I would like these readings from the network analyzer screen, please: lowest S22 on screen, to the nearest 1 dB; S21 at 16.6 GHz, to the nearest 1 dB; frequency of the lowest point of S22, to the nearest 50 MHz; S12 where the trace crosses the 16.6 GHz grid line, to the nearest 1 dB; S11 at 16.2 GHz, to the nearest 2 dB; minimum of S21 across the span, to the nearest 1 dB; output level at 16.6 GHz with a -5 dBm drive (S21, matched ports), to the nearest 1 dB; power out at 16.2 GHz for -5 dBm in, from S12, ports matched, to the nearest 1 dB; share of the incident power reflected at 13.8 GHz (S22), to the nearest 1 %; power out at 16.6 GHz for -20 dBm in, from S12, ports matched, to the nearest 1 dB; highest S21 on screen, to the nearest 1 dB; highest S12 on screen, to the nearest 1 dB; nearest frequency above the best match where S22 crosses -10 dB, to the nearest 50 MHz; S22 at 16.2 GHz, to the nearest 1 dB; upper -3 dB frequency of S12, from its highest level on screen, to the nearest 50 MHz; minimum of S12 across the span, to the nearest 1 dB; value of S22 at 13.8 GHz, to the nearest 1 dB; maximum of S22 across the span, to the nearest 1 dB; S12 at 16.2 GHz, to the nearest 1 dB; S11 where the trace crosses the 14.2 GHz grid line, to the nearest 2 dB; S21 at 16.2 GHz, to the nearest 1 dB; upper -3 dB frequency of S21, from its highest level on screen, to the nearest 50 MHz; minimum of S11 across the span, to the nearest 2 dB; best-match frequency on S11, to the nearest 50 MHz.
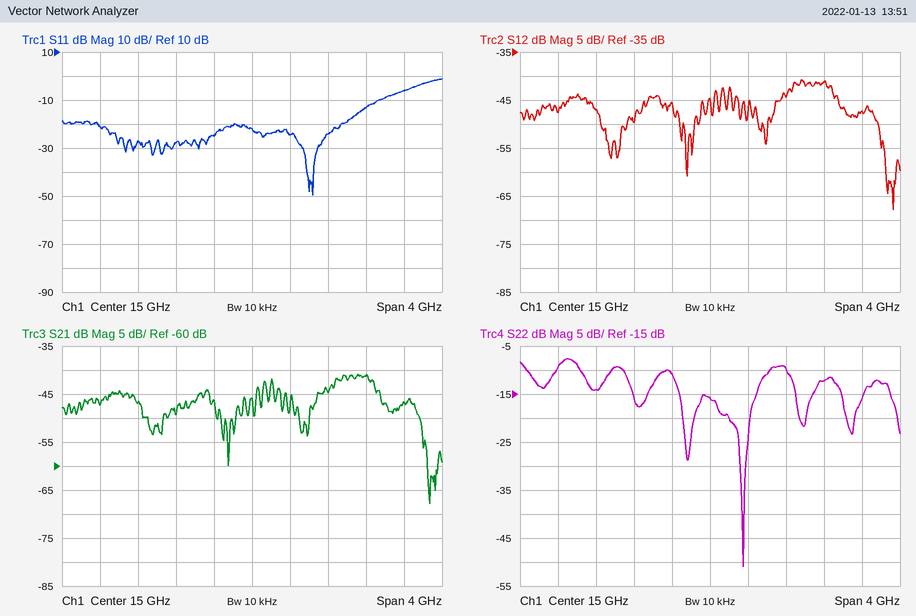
-51 dB
-47 dB
15.35 GHz
-47 dB
-14 dB
-68 dB
-52 dBm
-46 dBm
4 %
-67 dBm
-41 dB
-41 dB
15.65 GHz
-12 dB
16.30 GHz
-68 dB
-14 dB
-8 dB
-41 dB
-28 dB
-41 dB
16.30 GHz
-50 dB
15.65 GHz
